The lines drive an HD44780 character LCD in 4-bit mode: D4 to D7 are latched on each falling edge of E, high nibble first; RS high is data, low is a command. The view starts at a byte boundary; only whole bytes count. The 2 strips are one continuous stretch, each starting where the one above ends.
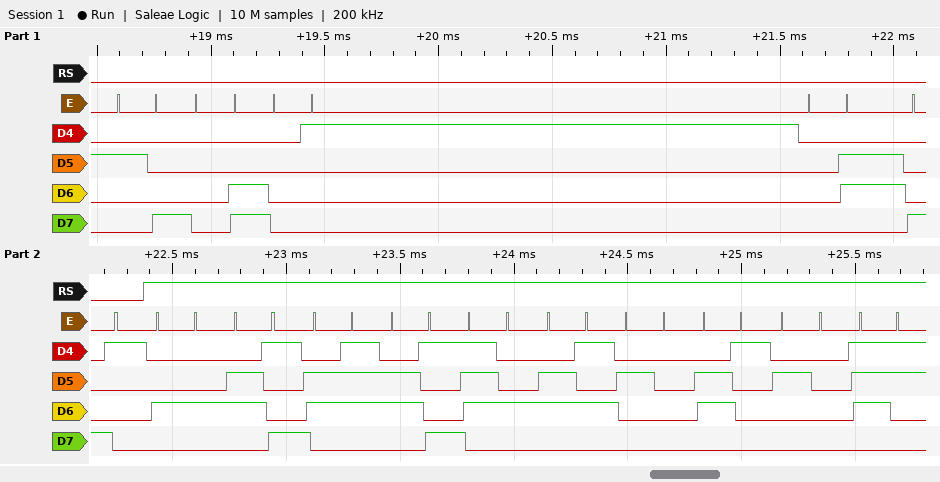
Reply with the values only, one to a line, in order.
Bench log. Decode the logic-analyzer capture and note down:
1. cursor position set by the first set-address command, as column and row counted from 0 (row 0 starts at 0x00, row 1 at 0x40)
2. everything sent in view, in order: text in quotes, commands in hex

column 1, row 0
0x28 0x0C 0x01 0x06 0x81 "Digite a s"
